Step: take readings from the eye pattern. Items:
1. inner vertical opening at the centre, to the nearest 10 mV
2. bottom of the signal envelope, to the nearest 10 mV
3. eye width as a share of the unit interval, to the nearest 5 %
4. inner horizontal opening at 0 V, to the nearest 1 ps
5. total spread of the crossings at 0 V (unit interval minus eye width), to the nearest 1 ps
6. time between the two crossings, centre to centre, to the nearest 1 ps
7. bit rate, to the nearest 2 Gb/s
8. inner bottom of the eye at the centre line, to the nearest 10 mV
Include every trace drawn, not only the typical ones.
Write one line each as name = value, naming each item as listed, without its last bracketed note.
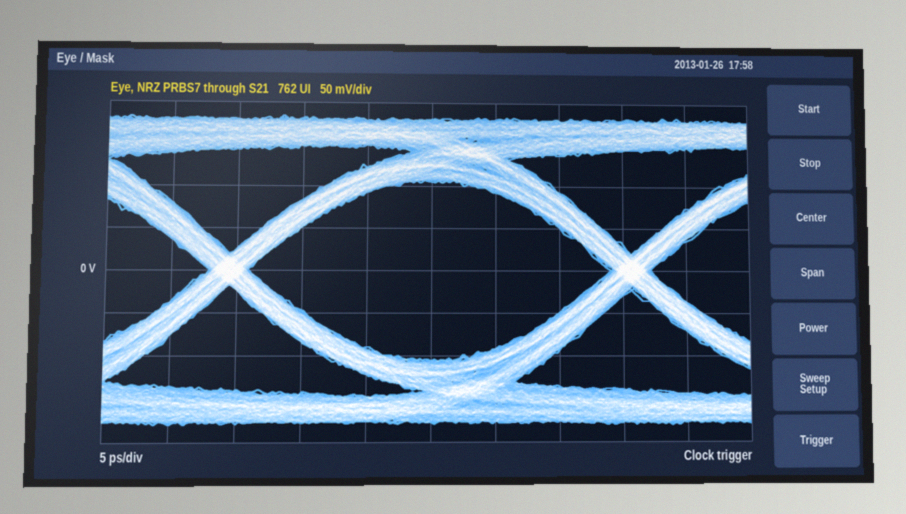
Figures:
inner vertical opening at the centre, to the nearest 10 mV = 210 mV
bottom of the signal envelope, to the nearest 10 mV = -180 mV
eye width as a share of the unit interval, to the nearest 5 % = 90 %
inner horizontal opening at 0 V, to the nearest 1 ps = 28 ps
total spread of the crossings at 0 V (unit interval minus eye width), to the nearest 1 ps = 3 ps
time between the two crossings, centre to centre, to the nearest 1 ps = 31 ps
bit rate, to the nearest 2 Gb/s = 32 Gb/s
inner bottom of the eye at the centre line, to the nearest 10 mV = -110 mV
